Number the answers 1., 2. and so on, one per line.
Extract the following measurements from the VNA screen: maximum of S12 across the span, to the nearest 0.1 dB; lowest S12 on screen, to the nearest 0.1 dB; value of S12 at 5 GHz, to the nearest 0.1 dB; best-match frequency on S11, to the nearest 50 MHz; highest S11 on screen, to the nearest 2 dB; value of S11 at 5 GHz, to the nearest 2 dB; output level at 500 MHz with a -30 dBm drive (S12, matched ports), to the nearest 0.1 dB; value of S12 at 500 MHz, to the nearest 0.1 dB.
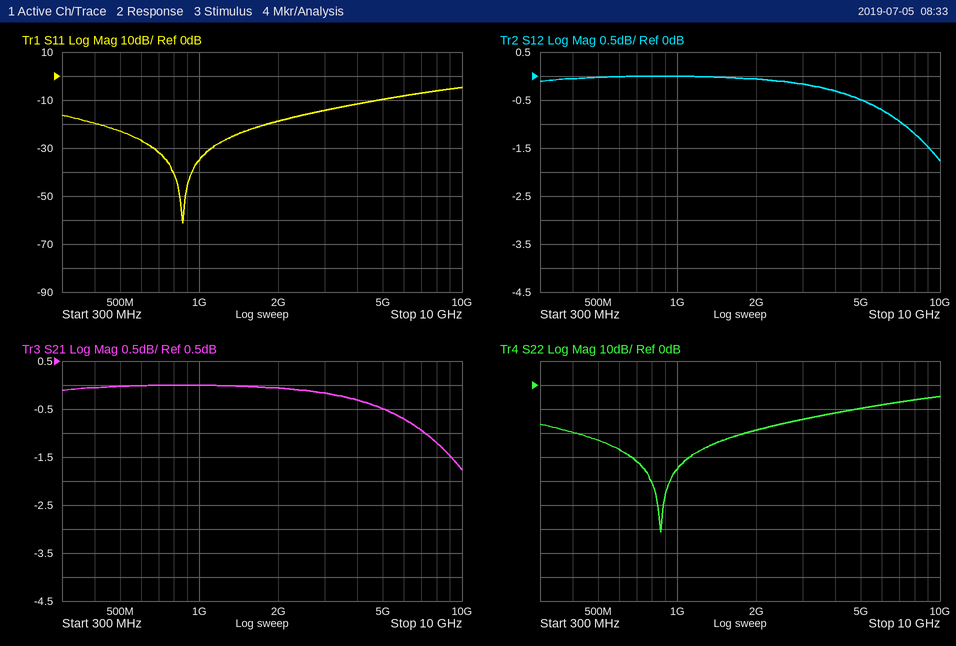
1. 0.0 dB
2. -1.8 dB
3. -0.5 dB
4. 850 MHz
5. -4 dB
6. -10 dB
7. -30.0 dBm
8. 0.0 dB
